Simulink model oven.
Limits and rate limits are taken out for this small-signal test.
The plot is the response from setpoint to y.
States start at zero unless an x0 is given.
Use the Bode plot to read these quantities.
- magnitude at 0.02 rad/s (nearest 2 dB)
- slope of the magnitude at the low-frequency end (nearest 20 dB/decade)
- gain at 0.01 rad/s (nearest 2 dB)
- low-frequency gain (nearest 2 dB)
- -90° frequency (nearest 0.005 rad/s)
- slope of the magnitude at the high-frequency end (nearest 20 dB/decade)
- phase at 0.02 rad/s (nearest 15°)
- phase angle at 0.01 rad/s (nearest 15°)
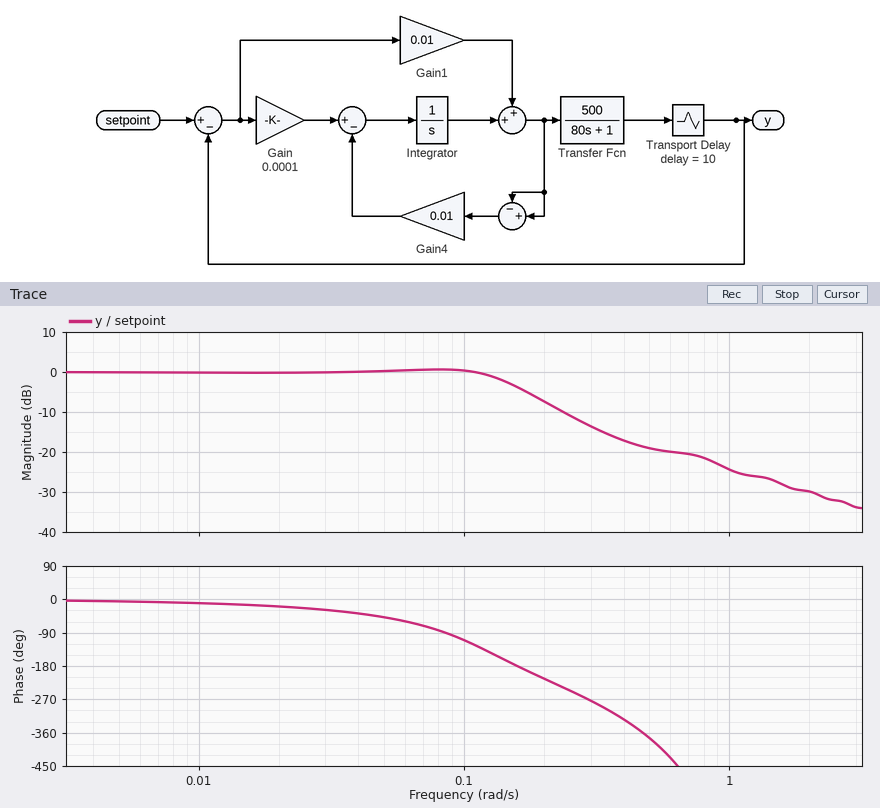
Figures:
0 dB
0 dB/decade
0 dB
0 dB
0.085 rad/s
-20 dB/decade
-15°
-15°
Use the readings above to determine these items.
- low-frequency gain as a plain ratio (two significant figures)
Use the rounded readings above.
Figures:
1.0
